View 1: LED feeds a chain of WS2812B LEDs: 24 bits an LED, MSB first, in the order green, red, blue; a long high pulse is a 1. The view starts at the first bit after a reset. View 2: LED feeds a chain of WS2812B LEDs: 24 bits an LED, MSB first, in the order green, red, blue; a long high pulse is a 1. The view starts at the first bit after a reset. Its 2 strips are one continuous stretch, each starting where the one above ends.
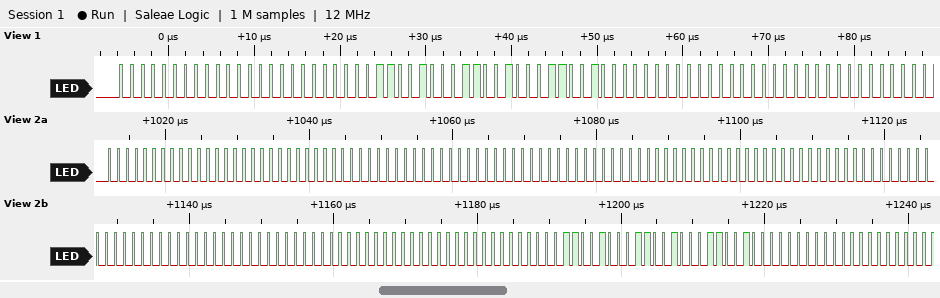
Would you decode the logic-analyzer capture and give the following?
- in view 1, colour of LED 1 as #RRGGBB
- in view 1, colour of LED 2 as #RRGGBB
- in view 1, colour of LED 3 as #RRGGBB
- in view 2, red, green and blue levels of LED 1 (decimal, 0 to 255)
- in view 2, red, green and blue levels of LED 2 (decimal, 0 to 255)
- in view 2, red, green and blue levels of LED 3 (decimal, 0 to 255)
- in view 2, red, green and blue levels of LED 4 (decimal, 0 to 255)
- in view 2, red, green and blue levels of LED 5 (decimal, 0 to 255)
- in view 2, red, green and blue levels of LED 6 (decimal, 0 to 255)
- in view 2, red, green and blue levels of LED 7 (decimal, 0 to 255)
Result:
#000000
#C8C8C8
#000000
0, 0, 0
0, 0, 0
0, 0, 0
0, 0, 0
0, 0, 0
0, 0, 0
200, 200, 200
